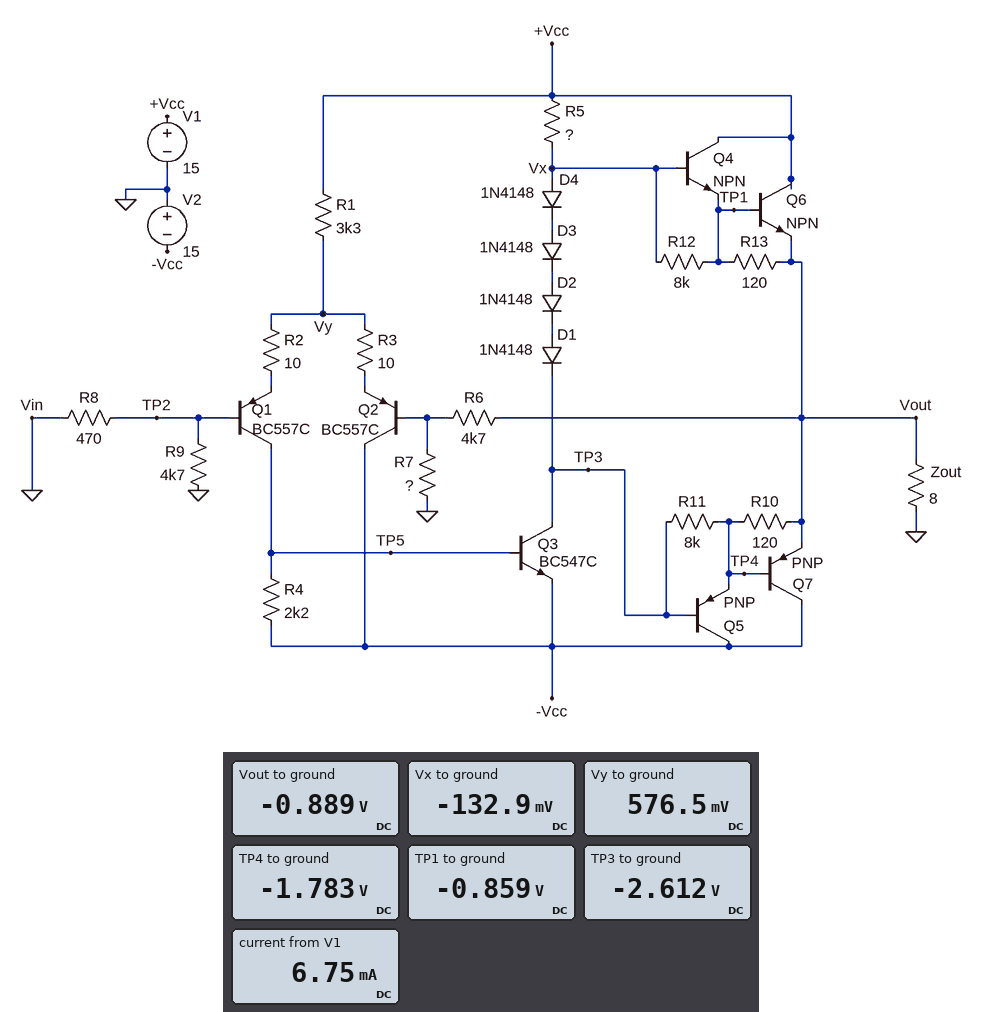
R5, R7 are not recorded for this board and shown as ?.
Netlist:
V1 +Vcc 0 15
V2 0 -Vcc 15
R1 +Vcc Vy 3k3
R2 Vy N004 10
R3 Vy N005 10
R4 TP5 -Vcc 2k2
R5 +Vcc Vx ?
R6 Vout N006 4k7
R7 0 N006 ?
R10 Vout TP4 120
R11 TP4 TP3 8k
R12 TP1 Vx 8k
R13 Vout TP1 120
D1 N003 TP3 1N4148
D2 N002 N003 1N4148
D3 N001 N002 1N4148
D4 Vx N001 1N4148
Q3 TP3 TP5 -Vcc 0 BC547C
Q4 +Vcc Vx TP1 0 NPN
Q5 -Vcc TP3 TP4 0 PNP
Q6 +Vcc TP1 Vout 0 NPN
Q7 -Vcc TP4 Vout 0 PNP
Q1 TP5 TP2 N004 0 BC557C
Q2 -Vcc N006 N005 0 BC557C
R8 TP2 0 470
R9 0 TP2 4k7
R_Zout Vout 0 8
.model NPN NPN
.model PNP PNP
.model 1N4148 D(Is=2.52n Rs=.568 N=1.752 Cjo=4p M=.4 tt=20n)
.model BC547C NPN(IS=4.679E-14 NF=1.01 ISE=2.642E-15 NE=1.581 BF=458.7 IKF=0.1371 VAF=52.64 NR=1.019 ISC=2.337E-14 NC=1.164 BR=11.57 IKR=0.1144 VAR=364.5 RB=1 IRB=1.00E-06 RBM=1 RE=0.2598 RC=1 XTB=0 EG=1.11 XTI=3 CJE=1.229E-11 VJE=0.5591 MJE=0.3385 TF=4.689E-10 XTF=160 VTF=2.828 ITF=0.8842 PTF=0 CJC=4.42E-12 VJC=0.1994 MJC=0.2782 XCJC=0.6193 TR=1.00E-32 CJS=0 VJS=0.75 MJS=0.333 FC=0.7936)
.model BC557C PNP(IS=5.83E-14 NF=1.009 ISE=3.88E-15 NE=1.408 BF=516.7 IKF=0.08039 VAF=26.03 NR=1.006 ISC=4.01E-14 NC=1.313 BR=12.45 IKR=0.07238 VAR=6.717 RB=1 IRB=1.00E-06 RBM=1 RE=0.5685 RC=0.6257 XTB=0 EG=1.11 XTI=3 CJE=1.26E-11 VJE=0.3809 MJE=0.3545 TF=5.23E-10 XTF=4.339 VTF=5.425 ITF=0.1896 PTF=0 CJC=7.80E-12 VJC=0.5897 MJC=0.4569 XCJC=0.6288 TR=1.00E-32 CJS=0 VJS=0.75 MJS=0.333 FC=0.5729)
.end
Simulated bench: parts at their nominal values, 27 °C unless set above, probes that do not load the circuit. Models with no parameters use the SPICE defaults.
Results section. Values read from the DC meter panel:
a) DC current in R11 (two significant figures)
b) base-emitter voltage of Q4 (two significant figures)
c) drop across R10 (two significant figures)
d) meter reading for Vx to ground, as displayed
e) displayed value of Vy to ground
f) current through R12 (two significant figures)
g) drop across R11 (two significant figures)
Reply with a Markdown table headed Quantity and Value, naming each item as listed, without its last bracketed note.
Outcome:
| Quantity | Value |
|---|---|
| DC current in R11 | 100 µA |
| base-emitter voltage of Q4 | 730 mV |
| drop across R10 | 890 mV |
| meter reading for Vx to ground, as displayed | -132.9 mV |
| displayed value of Vy to ground | 576.5 mV |
| current through R12 | 91 µA |
| drop across R11 | 830 mV |
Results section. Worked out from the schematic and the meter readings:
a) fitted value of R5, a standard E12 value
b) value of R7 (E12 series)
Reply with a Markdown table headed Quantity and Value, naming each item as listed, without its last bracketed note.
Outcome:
| Quantity | Value |
|---|---|
| fitted value of R5, a standard E12 value | 6.8 kΩ |
| value of R7 | 680 Ω |
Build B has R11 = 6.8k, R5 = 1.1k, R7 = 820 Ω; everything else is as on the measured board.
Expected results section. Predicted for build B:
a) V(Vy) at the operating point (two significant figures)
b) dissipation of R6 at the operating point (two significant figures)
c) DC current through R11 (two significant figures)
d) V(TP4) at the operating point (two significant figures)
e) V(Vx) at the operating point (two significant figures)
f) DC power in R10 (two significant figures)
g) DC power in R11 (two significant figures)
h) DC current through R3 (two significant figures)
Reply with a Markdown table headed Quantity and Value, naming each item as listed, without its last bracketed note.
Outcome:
| Quantity | Value |
|---|---|
| V(Vy) at the operating point | 580 mV |
| dissipation of R6 at the operating point | 82 µW |
| DC current through R11 | 120 µA |
| V(TP4) at the operating point | -1.6 V |
| V(Vx) at the operating point | 390 mV |
| DC power in R10 | 6.6 mW |
| DC power in R11 | 100 µW |
| DC current through R3 | 4.0 mA |
